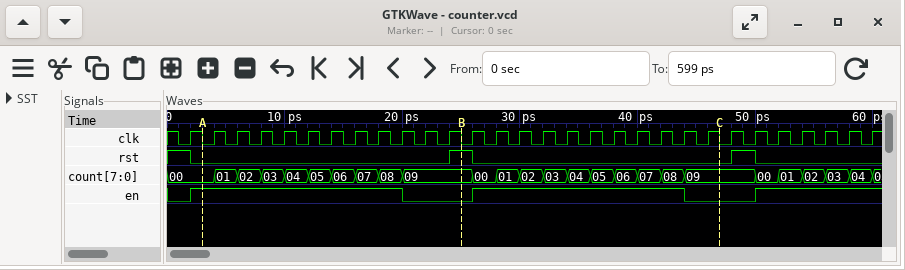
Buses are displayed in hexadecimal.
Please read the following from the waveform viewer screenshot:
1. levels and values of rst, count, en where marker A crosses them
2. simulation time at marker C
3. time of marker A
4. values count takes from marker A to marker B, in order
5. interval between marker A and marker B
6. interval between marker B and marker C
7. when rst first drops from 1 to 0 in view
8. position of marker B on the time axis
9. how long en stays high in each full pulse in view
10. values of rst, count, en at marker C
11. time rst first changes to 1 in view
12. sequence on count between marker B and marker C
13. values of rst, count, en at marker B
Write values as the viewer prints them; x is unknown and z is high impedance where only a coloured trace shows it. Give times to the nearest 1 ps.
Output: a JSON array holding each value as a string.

["rst=0, count=00, en=1", "47 ps", "3 ps", "00, 01, 02, 03, 04, 05, 06, 07, 08, 09", "22 ps", "22 ps", "2 ps", "25 ps", "18 ps, 18 ps", "rst=0, count=09, en=0", "24 ps", "09, 00, 01, 02, 03, 04, 05, 06, 07, 08, 09", "rst=1, count=09, en=0"]
